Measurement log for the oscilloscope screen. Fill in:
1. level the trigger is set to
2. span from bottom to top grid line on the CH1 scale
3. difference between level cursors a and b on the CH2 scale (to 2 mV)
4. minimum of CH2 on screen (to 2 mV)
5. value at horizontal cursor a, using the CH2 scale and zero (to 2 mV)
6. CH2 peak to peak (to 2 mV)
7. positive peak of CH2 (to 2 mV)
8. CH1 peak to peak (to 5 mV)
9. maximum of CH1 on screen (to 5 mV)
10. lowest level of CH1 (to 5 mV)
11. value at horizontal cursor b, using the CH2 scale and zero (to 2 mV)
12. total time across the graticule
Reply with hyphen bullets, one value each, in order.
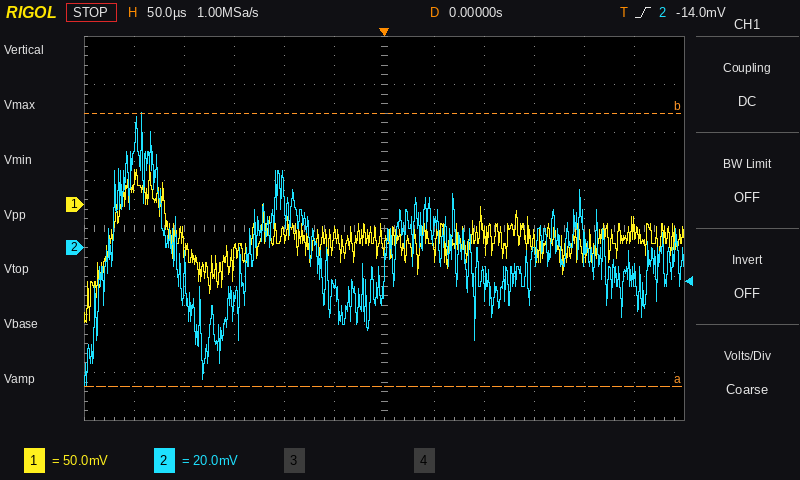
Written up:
- -14.0 mV
- 400 mV
- 114 mV
- -58 mV
- -58 mV
- 114 mV
- 56 mV
- 165 mV
- 40 mV
- -125 mV
- 56 mV
- 600 µs
